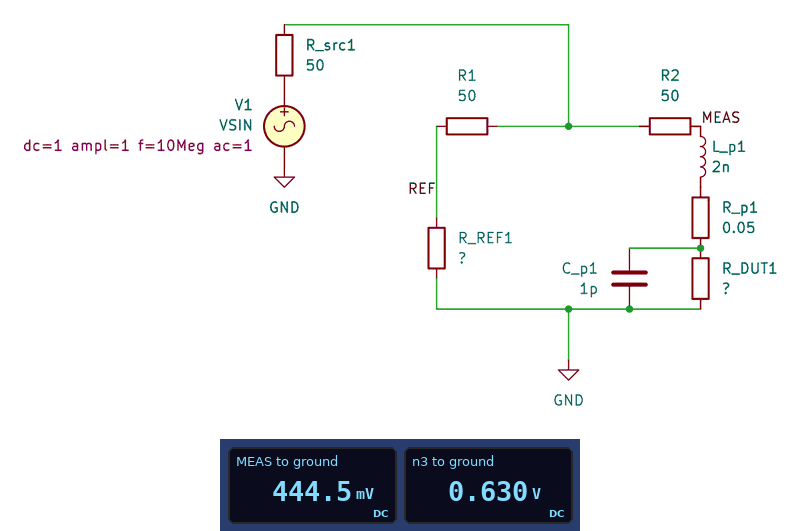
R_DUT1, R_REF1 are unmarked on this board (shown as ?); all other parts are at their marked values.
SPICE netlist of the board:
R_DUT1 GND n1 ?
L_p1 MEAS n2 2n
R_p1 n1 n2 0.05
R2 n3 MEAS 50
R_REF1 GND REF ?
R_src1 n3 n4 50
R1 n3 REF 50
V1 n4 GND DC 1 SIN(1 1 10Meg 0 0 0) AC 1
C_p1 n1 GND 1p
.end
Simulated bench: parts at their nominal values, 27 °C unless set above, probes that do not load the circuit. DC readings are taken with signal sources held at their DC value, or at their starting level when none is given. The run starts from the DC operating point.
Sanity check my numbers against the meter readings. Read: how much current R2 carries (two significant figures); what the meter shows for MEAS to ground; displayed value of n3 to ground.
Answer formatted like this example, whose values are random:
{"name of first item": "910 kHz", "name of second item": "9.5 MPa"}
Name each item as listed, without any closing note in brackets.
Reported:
{"how much current R2 carries": "3.7 mA", "what the meter shows for MEAS to ground": "444.5 mV", "displayed value of n3 to ground": "0.630 V"}
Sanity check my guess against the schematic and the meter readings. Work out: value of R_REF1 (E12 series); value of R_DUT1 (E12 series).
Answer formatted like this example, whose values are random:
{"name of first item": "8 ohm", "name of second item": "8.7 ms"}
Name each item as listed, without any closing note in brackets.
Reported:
{"value of R_REF1": "120 Ω", "value of R_DUT1": "120 Ω"}
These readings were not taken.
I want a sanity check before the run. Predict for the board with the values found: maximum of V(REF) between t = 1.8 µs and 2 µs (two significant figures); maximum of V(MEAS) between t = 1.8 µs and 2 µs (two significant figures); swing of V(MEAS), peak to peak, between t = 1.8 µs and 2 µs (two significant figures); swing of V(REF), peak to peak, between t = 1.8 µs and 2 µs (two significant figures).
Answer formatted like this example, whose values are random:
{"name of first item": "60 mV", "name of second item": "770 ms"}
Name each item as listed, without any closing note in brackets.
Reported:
{"maximum of V(REF) between t = 1.8 µs and 2 µs": "890 mV", "maximum of V(MEAS) between t = 1.8 µs and 2 µs": "890 mV", "swing of V(MEAS), peak to peak, between t = 1.8 µs and 2 µs": "890 mV", "swing of V(REF), peak to peak, between t = 1.8 µs and 2 µs": "890 mV"}
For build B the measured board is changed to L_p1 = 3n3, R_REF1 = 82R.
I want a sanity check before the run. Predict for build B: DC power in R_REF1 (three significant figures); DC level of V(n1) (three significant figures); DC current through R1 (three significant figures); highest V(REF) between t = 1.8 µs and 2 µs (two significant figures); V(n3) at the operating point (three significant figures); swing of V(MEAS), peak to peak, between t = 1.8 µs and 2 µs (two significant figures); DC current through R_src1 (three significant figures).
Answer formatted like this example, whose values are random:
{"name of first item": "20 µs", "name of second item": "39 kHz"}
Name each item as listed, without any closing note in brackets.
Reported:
{"DC power in R_REF1": "1.68 mW", "DC level of V(n1)": "422 mV", "DC current through R1": "4.53 mA", "highest V(REF) between t = 1.8 µs and 2 µs": "740 mV", "V(n3) at the operating point": "598 mV", "swing of V(MEAS), peak to peak, between t = 1.8 µs and 2 µs": "840 mV", "DC current through R_src1": "8.04 mA"}
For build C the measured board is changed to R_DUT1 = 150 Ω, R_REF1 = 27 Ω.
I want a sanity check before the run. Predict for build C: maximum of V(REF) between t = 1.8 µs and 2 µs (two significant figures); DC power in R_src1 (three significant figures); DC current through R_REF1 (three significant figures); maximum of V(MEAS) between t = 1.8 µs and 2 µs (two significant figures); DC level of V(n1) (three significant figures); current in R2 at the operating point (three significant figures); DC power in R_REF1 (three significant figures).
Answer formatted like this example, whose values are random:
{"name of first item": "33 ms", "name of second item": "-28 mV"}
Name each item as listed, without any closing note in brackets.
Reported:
{"maximum of V(REF) between t = 1.8 µs and 2 µs": "370 mV", "DC power in R_src1": "4.48 mW", "DC current through R_REF1": "6.84 mA", "maximum of V(MEAS) between t = 1.8 µs and 2 µs": "790 mV", "DC level of V(n1)": "395 mV", "current in R2 at the operating point": "2.63 mA", "DC power in R_REF1": "1.26 mW"}
